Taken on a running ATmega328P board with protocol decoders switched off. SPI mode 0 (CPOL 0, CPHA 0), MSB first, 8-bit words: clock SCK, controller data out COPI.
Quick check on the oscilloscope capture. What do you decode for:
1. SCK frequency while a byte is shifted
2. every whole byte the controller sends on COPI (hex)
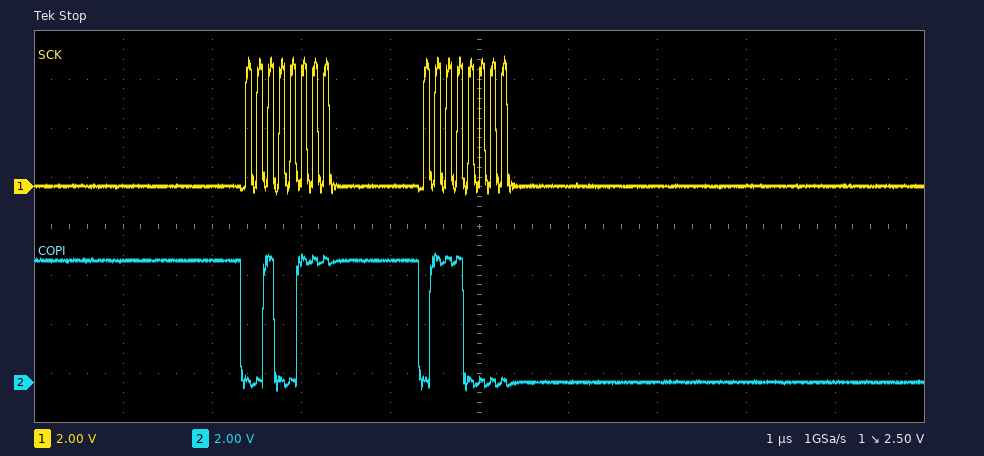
8 MHz
0x27 0x70
